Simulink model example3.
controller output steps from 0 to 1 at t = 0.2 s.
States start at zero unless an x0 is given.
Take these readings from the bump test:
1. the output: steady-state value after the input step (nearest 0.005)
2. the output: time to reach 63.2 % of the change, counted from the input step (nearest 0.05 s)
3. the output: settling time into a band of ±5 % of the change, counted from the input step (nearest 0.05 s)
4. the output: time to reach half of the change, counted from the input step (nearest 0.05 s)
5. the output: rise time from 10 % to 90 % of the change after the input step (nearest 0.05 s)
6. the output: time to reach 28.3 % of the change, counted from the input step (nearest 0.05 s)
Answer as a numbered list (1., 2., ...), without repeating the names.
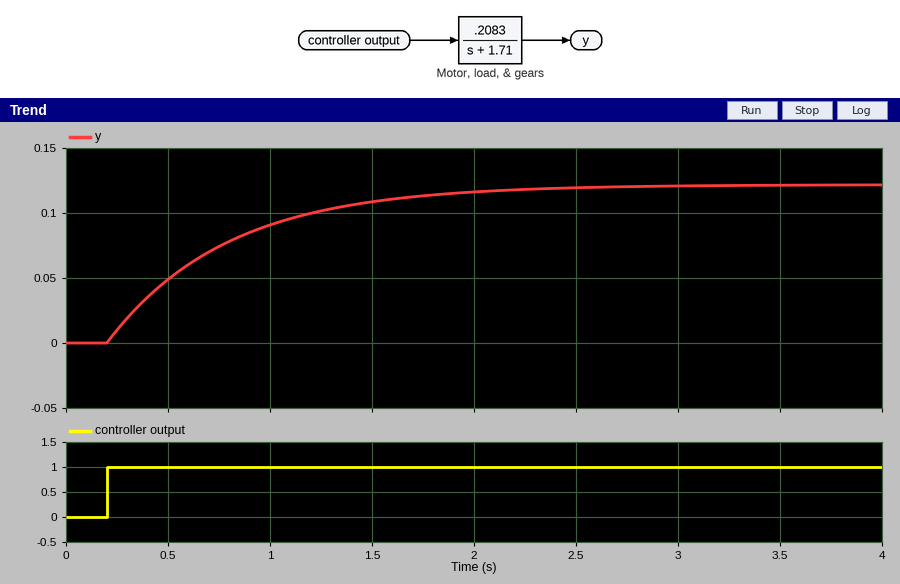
1. 0.120
2. 0.60 s
3. 1.75 s
4. 0.40 s
5. 1.30 s
6. 0.20 s
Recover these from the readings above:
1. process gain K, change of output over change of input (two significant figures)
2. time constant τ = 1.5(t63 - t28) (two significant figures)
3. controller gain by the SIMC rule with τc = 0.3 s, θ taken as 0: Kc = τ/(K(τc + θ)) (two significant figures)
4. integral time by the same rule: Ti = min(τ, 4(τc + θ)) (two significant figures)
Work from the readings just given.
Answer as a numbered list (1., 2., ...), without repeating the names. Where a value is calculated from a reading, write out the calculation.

1. (0.12 - 0) / 1 = 0.12
2. 1.5 × (0.6 - 0.2) = 0.60 s
3. 0.6 / (0.12 × (0.3 + 0)) = 17
4. min(0.6, 4 × (0.3 + 0)) = 0.60 s
